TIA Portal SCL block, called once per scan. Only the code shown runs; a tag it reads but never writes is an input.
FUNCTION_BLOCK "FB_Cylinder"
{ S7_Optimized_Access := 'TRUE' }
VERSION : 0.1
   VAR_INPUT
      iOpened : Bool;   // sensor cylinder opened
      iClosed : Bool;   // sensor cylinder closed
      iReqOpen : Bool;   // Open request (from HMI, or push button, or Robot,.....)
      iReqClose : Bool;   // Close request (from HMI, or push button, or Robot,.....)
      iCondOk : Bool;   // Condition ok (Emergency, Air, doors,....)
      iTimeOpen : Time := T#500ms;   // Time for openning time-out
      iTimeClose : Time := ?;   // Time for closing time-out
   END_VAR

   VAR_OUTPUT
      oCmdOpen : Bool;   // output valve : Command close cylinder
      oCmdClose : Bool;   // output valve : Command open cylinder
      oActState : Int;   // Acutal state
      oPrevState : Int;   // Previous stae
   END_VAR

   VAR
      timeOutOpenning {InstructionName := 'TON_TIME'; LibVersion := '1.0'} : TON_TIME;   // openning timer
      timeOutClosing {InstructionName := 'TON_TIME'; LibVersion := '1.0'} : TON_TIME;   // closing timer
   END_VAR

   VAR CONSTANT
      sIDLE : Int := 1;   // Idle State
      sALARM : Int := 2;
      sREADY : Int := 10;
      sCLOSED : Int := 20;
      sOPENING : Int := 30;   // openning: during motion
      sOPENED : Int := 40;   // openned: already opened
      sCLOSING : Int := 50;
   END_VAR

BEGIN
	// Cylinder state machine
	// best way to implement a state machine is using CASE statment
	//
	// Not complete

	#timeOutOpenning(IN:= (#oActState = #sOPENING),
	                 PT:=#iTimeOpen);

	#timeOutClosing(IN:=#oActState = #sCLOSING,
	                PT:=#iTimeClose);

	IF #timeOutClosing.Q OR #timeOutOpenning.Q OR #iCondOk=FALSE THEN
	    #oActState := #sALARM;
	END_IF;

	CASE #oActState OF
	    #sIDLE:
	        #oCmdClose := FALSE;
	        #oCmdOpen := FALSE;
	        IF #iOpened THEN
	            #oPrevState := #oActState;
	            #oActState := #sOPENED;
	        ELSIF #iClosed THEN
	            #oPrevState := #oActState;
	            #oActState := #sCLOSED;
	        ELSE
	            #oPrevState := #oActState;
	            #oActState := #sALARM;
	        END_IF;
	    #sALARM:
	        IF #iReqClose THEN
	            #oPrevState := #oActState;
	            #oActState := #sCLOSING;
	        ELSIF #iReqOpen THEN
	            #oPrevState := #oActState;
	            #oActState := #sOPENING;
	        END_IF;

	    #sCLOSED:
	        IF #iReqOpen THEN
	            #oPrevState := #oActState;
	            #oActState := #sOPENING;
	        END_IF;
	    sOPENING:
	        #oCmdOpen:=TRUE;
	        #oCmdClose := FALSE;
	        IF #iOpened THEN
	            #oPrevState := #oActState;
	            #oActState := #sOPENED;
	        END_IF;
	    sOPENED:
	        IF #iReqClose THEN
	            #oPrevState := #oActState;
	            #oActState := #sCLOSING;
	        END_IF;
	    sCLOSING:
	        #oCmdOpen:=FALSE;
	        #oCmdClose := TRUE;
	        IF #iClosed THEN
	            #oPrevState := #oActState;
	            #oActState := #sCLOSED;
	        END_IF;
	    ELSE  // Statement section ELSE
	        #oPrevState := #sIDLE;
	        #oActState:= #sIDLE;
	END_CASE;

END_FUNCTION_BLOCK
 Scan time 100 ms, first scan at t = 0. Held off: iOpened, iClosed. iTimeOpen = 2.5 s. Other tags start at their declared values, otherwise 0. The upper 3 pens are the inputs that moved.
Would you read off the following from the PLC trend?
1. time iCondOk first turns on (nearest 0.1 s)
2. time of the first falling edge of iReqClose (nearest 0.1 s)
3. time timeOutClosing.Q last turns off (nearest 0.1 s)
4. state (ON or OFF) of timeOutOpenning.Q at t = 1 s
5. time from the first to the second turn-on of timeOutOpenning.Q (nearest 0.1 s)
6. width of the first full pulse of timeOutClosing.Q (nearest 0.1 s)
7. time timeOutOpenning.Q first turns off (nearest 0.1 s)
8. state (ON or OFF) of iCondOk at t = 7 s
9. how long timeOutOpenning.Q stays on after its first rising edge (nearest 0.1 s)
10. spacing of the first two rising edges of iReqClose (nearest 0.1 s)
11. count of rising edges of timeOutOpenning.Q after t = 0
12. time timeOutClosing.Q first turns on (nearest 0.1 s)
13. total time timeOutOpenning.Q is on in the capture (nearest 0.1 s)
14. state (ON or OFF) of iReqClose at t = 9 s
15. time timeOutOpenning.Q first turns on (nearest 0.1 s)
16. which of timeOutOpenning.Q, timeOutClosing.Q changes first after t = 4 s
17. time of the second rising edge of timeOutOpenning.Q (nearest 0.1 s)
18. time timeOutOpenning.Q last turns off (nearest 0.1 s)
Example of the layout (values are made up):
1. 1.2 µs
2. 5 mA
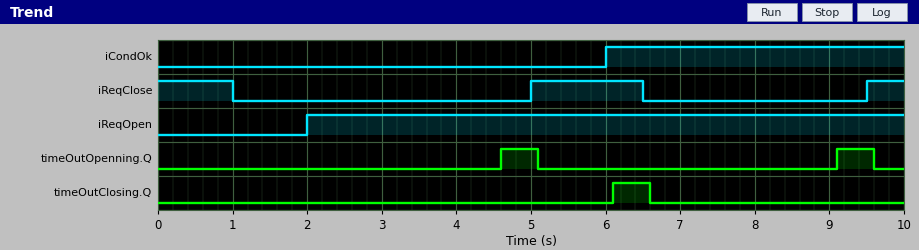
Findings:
1. 6.0 s
2. 1.0 s
3. 6.6 s
4. OFF
5. 4.5 s
6. 0.5 s
7. 5.1 s
8. ON
9. 0.5 s
10. 4.5 s
11. 2
12. 6.1 s
13. 1.0 s
14. OFF
15. 4.6 s
16. timeOutOpenning.Q
17. 9.1 s
18. 9.6 s
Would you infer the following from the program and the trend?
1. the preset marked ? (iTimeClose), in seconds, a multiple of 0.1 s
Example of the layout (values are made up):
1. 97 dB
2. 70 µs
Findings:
1. 1.0 s
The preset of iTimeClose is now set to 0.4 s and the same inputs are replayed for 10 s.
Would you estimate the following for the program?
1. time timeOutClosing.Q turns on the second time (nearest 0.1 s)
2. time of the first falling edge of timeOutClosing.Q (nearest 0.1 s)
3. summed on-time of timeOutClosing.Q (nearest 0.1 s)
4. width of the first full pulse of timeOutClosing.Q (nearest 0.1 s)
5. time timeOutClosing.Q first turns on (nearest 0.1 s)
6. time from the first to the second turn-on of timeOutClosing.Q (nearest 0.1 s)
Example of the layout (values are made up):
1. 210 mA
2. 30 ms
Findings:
1. 5.5 s
2. 1.1 s
3. 1.7 s
4. 0.6 s
5. 0.5 s
6. 5.0 s
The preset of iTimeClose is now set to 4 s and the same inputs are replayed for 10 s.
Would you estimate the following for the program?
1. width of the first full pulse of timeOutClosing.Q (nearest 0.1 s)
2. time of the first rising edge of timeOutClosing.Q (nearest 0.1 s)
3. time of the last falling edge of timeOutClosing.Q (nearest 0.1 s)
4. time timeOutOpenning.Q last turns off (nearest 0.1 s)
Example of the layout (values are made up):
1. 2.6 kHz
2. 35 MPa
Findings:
1. 0.1 s
2. 9.1 s
3. 9.2 s
4. 5.1 s
